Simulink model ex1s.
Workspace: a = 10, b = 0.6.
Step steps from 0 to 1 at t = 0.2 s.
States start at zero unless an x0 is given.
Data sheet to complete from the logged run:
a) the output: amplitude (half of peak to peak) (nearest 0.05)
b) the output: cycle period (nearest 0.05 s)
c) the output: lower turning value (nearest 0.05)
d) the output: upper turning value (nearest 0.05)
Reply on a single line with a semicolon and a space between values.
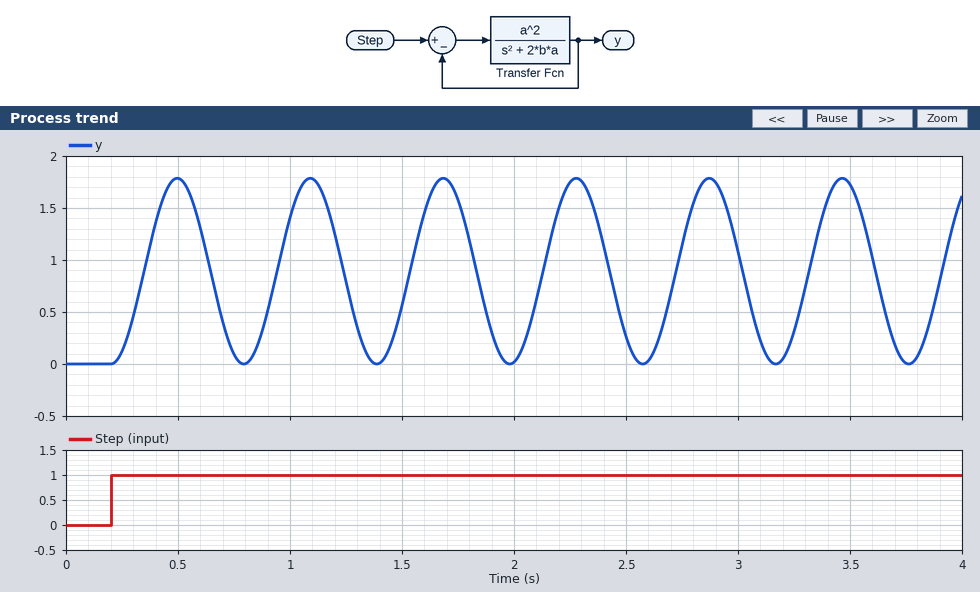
0.90; 0.60 s; 0.00; 1.80
